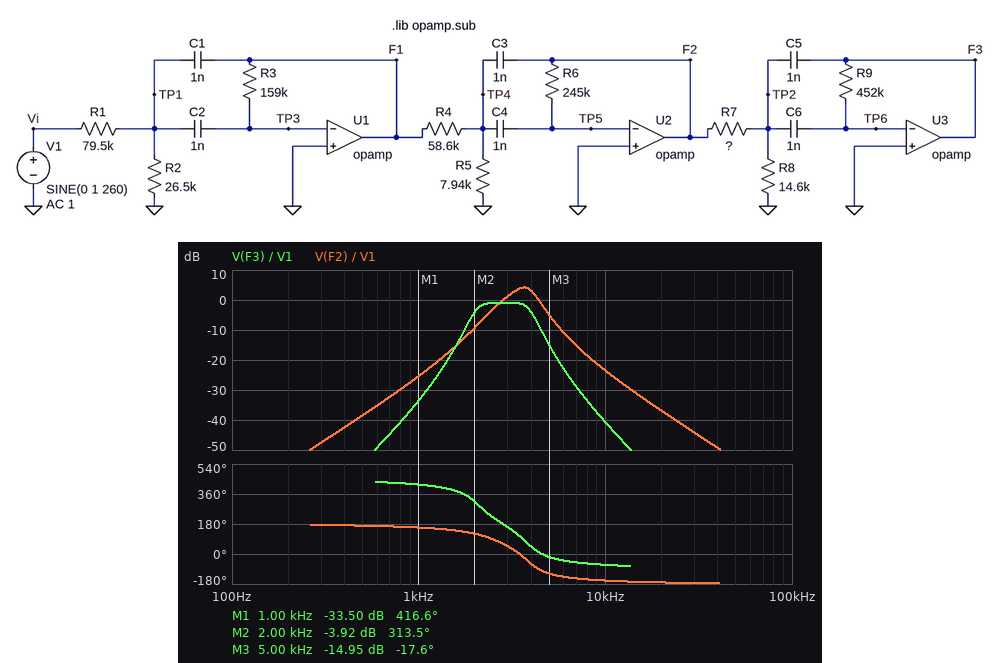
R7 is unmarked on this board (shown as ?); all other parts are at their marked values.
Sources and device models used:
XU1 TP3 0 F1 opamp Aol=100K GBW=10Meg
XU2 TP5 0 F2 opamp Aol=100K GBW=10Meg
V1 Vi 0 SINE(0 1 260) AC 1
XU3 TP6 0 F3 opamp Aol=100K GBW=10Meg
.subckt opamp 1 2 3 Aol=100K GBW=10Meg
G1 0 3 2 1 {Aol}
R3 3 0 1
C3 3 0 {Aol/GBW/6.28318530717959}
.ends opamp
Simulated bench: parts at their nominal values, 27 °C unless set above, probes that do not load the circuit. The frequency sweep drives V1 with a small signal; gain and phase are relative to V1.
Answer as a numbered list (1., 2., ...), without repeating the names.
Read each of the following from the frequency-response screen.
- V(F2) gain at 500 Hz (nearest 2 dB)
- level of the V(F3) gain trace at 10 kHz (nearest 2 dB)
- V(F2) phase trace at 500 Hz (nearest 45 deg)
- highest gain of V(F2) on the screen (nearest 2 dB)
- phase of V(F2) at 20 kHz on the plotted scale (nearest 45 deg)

1. -38 dB
2. -40 dB
3. 180 deg
4. 4 dB
5. -180 deg
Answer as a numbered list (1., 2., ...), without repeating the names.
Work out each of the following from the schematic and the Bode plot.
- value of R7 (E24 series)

1. 120 kΩ
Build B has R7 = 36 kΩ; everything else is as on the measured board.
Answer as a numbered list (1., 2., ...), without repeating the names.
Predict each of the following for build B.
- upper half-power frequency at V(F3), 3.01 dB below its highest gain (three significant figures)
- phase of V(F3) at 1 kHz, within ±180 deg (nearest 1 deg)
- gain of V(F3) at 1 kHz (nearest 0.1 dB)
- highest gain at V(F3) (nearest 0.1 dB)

1. 3.81 kHz
2. 60 deg
3. -25.4 dB
4. 12.0 dB
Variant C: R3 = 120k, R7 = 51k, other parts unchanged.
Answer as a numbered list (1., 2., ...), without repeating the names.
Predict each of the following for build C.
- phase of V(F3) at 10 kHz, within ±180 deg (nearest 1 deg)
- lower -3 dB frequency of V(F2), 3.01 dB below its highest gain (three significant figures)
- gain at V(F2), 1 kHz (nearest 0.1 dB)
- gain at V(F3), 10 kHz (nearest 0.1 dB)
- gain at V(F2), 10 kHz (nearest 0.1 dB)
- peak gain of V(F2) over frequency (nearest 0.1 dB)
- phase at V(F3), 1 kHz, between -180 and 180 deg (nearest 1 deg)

1. -61 deg
2. 3.18 kHz
3. -28.1 dB
4. -33.1 dB
5. -23.4 dB
6. 3.4 dB
7. 59 deg
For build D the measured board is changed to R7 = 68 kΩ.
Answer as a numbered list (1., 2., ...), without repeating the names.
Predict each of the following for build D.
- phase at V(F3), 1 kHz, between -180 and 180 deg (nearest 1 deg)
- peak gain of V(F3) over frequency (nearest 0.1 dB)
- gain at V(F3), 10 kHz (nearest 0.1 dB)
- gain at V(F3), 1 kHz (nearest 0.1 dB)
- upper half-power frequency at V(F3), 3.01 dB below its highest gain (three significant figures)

1. 58 deg
2. 4.8 dB
3. -35.7 dB
4. -29.4 dB
5. 3.94 kHz
